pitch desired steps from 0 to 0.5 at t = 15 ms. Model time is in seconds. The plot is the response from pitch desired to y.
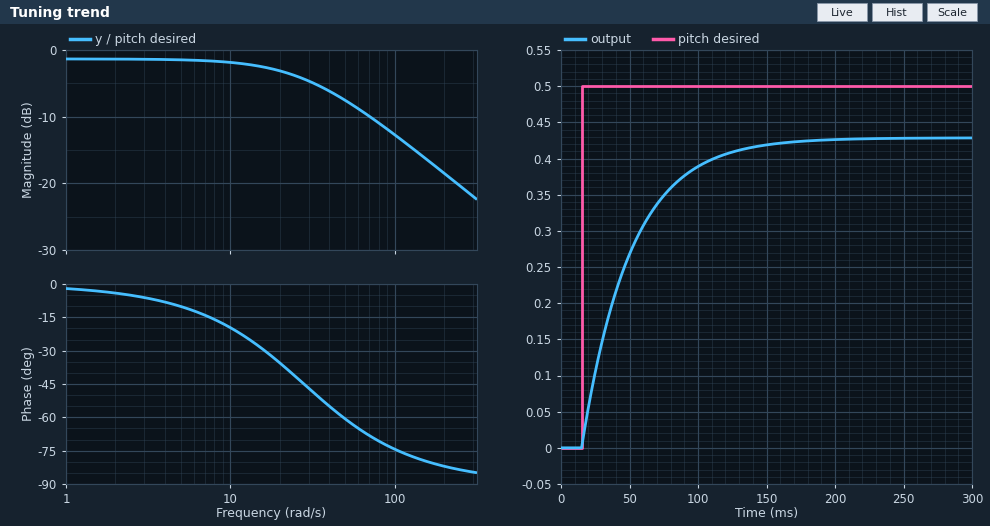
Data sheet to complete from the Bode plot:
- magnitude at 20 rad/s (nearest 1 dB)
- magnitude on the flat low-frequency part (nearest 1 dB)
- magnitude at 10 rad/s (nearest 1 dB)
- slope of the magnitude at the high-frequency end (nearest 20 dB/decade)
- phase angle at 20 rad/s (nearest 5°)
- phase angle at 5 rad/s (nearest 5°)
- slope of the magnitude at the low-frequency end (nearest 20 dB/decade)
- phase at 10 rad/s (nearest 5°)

-3 dB
-1 dB
-2 dB
-20 dB/decade
-35°
-10°
0 dB/decade
-20°
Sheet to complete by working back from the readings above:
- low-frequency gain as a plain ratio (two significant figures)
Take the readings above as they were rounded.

0.89
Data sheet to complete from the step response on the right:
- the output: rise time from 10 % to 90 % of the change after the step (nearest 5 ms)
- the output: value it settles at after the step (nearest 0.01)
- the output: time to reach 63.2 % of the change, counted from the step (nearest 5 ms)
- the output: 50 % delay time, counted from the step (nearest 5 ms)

80 ms
0.43
35 ms
25 ms
